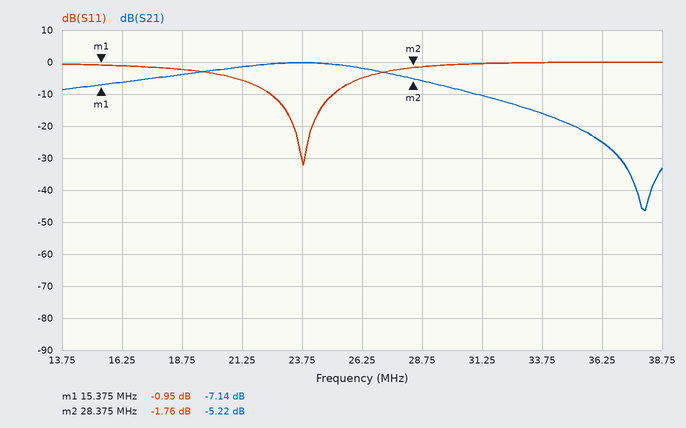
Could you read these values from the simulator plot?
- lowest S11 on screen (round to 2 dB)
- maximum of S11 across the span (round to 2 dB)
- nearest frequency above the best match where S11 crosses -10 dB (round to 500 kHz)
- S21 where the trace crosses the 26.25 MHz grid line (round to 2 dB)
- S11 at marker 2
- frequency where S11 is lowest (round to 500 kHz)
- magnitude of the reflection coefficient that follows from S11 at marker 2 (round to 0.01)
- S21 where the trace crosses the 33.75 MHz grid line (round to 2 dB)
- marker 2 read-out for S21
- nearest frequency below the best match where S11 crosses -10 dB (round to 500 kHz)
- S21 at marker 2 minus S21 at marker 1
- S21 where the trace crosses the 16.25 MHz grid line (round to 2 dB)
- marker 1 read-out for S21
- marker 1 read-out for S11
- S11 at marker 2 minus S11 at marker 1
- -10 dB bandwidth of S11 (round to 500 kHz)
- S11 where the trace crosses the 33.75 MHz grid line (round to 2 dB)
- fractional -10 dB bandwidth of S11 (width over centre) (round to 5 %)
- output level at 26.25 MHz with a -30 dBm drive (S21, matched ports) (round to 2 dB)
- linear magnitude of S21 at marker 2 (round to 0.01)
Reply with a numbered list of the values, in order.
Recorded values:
1. -32 dB
2. 0 dB
3. 25.0 MHz
4. -2 dB
5. -1.76 dB
6. 24.0 MHz
7. 0.82
8. -16 dB
9. -5.22 dB
10. 22.5 MHz
11. 1.92 dB
12. -6 dB
13. -7.14 dB
14. -0.95 dB
15. -0.81 dB
16. 2.5 MHz
17. 0 dB
18. 10 %
19. -32 dBm
20. 0.55
